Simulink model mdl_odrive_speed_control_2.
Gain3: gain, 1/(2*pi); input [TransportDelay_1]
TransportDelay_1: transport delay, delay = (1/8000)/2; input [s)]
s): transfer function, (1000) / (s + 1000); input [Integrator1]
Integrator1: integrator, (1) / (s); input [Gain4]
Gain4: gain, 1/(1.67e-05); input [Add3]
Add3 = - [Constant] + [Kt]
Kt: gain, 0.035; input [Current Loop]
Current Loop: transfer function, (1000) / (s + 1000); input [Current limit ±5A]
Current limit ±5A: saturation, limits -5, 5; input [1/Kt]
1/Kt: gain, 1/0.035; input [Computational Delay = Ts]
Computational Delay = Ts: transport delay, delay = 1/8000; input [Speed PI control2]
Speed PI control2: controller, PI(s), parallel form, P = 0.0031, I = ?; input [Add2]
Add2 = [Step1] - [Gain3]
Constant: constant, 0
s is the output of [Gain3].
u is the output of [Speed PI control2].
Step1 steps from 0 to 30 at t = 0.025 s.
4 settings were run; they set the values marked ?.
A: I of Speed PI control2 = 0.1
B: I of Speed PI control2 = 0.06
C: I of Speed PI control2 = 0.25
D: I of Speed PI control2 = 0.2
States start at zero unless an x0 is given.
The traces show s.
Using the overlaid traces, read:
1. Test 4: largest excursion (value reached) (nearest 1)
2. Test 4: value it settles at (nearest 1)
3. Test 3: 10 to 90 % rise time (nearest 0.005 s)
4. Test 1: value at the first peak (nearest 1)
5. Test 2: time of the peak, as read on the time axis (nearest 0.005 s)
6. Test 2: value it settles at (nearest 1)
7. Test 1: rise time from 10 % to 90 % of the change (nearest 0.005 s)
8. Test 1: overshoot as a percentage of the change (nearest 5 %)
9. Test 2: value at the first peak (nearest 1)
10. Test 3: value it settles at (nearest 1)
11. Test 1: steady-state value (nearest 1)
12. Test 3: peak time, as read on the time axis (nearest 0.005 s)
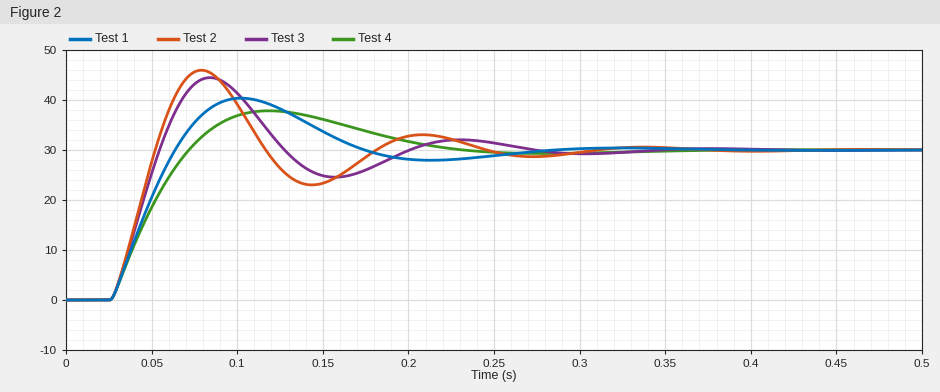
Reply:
38
30
0.020 s
40
0.080 s
30
0.030 s
35 %
46
30
30
0.085 s
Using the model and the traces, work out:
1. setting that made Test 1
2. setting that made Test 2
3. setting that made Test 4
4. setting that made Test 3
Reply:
A
C
B
D
